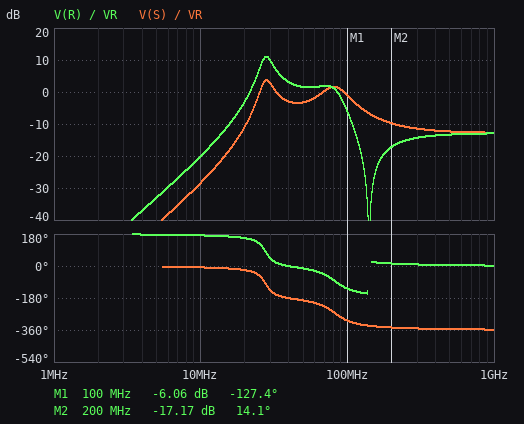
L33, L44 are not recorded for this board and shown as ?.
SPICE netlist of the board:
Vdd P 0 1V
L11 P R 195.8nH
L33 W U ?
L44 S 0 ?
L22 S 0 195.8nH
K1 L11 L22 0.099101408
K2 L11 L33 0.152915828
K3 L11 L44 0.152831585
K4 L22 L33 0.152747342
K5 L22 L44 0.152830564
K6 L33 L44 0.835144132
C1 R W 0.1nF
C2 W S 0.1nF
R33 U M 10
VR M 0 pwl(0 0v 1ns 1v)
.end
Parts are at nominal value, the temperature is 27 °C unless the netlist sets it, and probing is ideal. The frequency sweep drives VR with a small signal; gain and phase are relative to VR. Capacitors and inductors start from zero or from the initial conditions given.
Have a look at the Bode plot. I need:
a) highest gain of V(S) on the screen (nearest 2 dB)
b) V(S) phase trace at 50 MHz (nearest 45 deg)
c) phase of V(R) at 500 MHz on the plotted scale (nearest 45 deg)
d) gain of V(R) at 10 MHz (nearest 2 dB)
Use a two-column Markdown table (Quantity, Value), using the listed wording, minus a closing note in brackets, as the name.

| Quantity | Value |
|---|---|
| highest gain of V(S) on the screen | 4 dB |
| V(S) phase trace at 50 MHz | -180 deg |
| phase of V(R) at 500 MHz on the plotted scale | 0 deg |
| gain of V(R) at 10 MHz | -20 dB |
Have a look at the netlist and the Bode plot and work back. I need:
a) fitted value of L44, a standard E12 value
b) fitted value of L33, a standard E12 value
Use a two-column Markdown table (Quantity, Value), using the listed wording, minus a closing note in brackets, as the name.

| Quantity | Value |
|---|---|
| fitted value of L44, a standard E12 value | 120 nH |
| fitted value of L33, a standard E12 value | 120 nH |
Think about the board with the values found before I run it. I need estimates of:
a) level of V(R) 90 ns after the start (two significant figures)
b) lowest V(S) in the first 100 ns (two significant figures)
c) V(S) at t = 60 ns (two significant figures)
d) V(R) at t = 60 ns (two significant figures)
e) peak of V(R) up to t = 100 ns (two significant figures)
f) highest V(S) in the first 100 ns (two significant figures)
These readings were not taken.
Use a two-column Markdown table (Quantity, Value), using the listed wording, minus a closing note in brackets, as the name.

| Quantity | Value |
|---|---|
| level of V(R) 90 ns after the start | 990 mV |
| lowest V(S) in the first 100 ns | -360 mV |
| V(S) at t = 60 ns | 29 mV |
| V(R) at t = 60 ns | 930 mV |
| peak of V(R) up to t = 100 ns | 1.4 V |
| highest V(S) in the first 100 ns | 490 mV |
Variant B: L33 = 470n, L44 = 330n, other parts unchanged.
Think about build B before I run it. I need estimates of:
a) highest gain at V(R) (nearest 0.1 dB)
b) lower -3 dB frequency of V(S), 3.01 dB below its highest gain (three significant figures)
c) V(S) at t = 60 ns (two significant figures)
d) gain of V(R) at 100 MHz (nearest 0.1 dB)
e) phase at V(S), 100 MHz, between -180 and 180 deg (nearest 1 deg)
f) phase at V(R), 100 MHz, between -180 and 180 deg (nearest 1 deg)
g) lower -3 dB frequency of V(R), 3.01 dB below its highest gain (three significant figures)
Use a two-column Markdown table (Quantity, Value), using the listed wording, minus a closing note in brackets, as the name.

| Quantity | Value |
|---|---|
| highest gain at V(R) | 10.8 dB |
| lower -3 dB frequency of V(S), 3.01 dB below its highest gain | 48.5 MHz |
| V(S) at t = 60 ns | 83 mV |
| gain of V(R) at 100 MHz | -16.6 dB |
| phase at V(S), 100 MHz, between -180 and 180 deg | 8 deg |
| phase at V(R), 100 MHz, between -180 and 180 deg | -172 deg |
| lower -3 dB frequency of V(R), 3.01 dB below its highest gain | 48.4 MHz |
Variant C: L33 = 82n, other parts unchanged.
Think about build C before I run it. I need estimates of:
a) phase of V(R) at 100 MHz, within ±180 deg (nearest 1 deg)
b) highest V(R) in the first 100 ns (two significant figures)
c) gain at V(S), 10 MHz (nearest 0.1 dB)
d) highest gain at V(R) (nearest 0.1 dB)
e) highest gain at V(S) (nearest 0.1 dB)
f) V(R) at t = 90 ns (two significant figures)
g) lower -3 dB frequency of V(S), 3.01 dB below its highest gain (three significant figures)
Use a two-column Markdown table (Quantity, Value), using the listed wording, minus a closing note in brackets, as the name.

| Quantity | Value |
|---|---|
| phase of V(R) at 100 MHz, within ±180 deg | -113 deg |
| highest V(R) in the first 100 ns | 1.3 V |
| gain at V(S), 10 MHz | -31.6 dB |
| highest gain at V(R) | 12.1 dB |
| highest gain at V(S) | 3.9 dB |
| V(R) at t = 90 ns | 960 mV |
| lower -3 dB frequency of V(S), 3.01 dB below its highest gain | 27.7 MHz |
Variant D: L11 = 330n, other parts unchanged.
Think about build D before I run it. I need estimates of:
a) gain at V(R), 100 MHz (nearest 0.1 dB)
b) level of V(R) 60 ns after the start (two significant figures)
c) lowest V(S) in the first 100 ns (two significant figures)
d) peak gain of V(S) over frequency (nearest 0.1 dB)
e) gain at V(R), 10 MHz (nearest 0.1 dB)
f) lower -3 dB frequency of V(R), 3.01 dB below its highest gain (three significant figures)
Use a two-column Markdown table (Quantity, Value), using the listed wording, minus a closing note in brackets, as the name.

| Quantity | Value |
|---|---|
| gain at V(R), 100 MHz | -5.5 dB |
| level of V(R) 60 ns after the start | 1.0 V |
| lowest V(S) in the first 100 ns | -290 mV |
| peak gain of V(S) over frequency | 2.9 dB |
| gain at V(R), 10 MHz | -15.1 dB |
| lower -3 dB frequency of V(R), 3.01 dB below its highest gain | 21.6 MHz |
